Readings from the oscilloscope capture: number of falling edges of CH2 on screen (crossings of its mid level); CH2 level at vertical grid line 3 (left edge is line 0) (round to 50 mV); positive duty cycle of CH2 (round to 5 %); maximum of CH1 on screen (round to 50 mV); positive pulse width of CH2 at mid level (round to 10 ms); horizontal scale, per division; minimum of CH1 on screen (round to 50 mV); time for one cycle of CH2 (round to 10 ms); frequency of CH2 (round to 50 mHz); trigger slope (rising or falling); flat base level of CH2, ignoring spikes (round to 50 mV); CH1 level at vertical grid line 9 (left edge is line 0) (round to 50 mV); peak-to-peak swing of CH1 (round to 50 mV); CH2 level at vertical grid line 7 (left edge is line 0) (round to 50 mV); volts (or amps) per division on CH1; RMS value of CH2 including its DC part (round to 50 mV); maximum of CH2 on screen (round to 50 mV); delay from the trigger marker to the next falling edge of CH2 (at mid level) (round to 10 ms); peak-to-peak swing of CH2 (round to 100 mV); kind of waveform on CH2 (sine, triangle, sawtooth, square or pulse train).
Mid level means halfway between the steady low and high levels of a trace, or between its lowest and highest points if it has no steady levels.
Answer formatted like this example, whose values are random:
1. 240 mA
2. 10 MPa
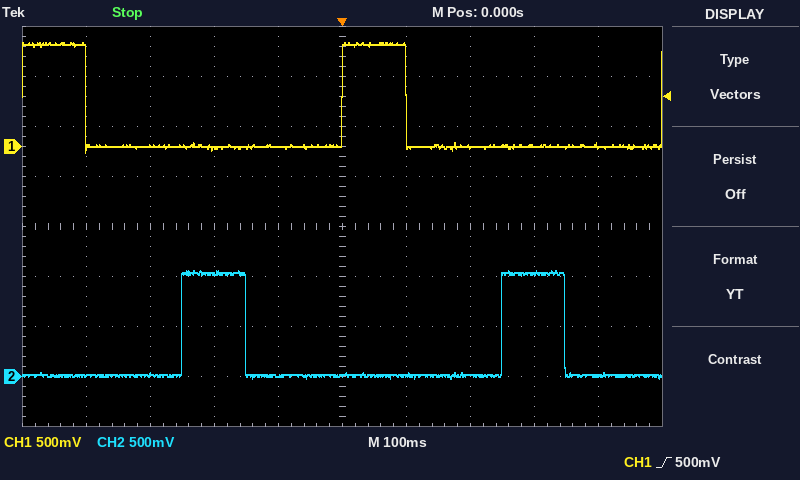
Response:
1. 2
2. 1.05 V
3. 20 %
4. 1.05 V
5. 100 ms
6. 100 ms
7. -50 mV
8. 500 ms
9. 2.00 Hz
10. rising
11. 0 mV
12. 0 mV
13. 1.10 V
14. 0 mV
15. 500 mV
16. 450 mV
17. 1.05 V
18. 350 ms
19. 1.10 V
20. pulse train
